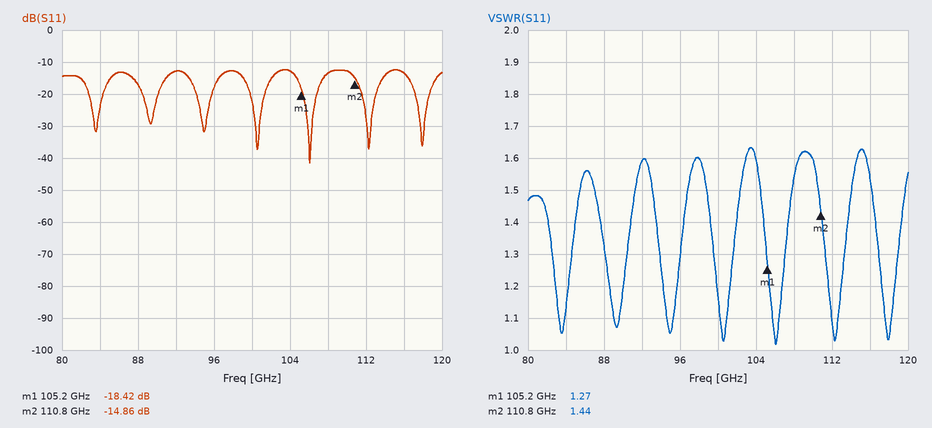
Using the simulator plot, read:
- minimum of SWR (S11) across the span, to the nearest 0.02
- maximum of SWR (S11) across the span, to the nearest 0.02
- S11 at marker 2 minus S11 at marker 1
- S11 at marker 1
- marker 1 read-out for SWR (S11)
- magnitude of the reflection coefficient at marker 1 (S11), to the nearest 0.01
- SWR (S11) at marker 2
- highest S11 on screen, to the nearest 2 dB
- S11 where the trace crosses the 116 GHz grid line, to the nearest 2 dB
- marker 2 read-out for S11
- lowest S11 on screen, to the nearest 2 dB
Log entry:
1.02
1.64
3.56 dB
-18.42 dB
1.27
0.12
1.44
-12 dB
-14 dB
-14.86 dB
-42 dB
